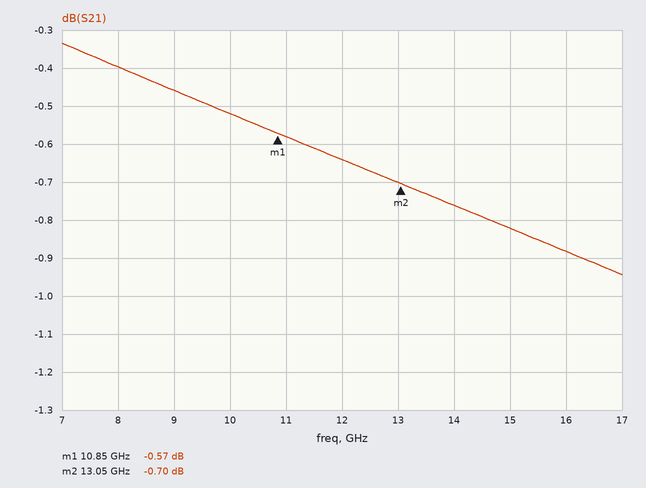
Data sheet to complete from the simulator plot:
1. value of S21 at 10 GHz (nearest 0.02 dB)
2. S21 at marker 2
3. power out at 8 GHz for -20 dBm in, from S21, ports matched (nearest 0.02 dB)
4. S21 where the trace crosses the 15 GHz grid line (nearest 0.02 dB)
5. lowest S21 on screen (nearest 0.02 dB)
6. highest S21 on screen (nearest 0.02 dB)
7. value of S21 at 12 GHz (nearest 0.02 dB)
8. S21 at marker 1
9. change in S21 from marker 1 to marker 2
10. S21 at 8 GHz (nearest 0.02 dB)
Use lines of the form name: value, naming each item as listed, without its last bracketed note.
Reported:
value of S21 at 10 GHz: -0.52 dB
S21 at marker 2: -0.70 dB
power out at 8 GHz for -20 dBm in, from S21, ports matched: -20.40 dBm
S21 where the trace crosses the 15 GHz grid line: -0.82 dB
lowest S21 on screen: -0.94 dB
highest S21 on screen: -0.34 dB
value of S21 at 12 GHz: -0.64 dB
S21 at marker 1: -0.57 dB
change in S21 from marker 1 to marker 2: -0.13 dB
S21 at 8 GHz: -0.40 dB
